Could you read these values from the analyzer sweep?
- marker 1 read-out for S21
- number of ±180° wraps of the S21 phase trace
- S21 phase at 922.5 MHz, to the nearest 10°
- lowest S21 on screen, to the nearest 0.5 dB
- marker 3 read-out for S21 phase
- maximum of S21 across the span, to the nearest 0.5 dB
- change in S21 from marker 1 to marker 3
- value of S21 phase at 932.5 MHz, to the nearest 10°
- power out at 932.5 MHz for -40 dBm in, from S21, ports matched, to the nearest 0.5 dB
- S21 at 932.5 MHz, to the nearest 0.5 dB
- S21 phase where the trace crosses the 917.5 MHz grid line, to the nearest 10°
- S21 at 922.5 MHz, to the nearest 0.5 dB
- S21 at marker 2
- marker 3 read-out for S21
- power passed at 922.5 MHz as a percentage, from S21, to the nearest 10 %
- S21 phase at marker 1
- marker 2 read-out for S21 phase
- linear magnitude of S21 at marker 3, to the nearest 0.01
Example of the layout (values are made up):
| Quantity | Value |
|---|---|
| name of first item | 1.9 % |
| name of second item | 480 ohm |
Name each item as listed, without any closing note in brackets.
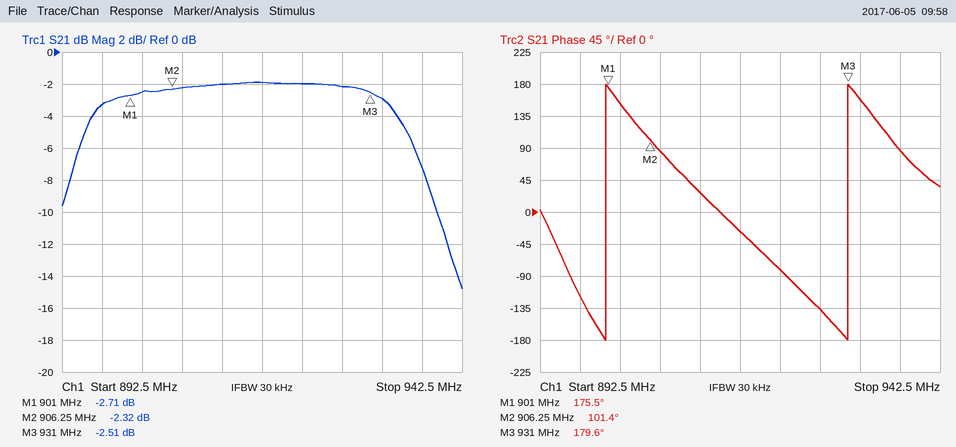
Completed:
| Quantity | Value |
|---|---|
| marker 1 read-out for S21 | -2.71 dB |
| number of ±180° wraps of the S21 phase trace | 2 |
| S21 phase at 922.5 MHz, to the nearest 10° | -80° |
| lowest S21 on screen, to the nearest 0.5 dB | -15.0 dB |
| marker 3 read-out for S21 phase | 179.6° |
| maximum of S21 across the span, to the nearest 0.5 dB | -2.0 dB |
| change in S21 from marker 1 to marker 3 | 0.20 dB |
| value of S21 phase at 932.5 MHz, to the nearest 10° | 160° |
| power out at 932.5 MHz for -40 dBm in, from S21, ports matched, to the nearest 0.5 dB | -43.0 dBm |
| S21 at 932.5 MHz, to the nearest 0.5 dB | -3.0 dB |
| S21 phase where the trace crosses the 917.5 MHz grid line, to the nearest 10° | -30° |
| S21 at 922.5 MHz, to the nearest 0.5 dB | -2.0 dB |
| S21 at marker 2 | -2.32 dB |
| marker 3 read-out for S21 | -2.51 dB |
| power passed at 922.5 MHz as a percentage, from S21, to the nearest 10 % | 60 % |
| S21 phase at marker 1 | 175.5° |
| marker 2 read-out for S21 phase | 101.4° |
| linear magnitude of S21 at marker 3, to the nearest 0.01 | 0.75 |
